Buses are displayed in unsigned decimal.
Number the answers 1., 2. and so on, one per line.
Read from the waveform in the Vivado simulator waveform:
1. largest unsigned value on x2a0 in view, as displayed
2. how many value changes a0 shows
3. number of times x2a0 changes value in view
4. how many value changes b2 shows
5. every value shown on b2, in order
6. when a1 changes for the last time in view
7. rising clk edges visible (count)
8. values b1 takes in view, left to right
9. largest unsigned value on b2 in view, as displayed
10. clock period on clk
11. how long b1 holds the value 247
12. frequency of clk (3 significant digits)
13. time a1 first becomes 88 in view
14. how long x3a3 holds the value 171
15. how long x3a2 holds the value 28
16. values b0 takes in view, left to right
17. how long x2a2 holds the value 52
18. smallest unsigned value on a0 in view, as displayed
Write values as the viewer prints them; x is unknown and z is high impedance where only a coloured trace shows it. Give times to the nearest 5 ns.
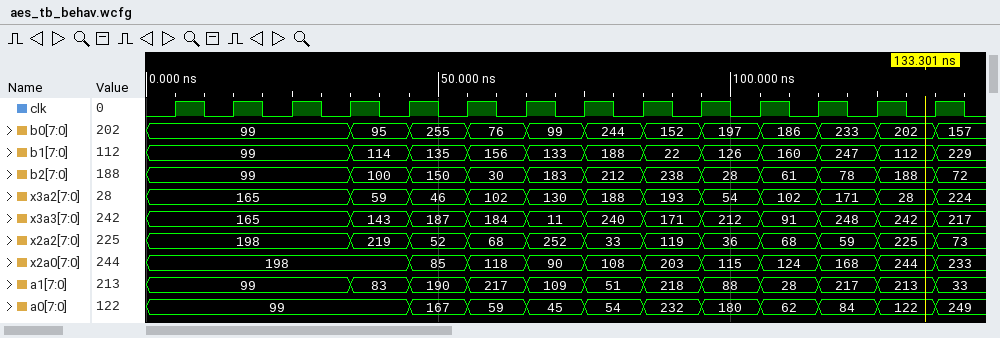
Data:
1. 244
2. 10
3. 10
4. 11
5. 99, 100, 150, 30, 183, 212, 238, 28, 61, 78, 188, 72
6. 135 ns
7. 14
8. 99, 114, 135, 156, 133, 188, 22, 126, 160, 247, 112, 229
9. 238
10. 10 ns
11. 10 ns
12. 100 MHz
13. 95 ns
14. 10 ns
15. 10 ns
16. 99, 95, 255, 76, 99, 244, 152, 197, 186, 233, 202, 157
17. 10 ns
18. 45
